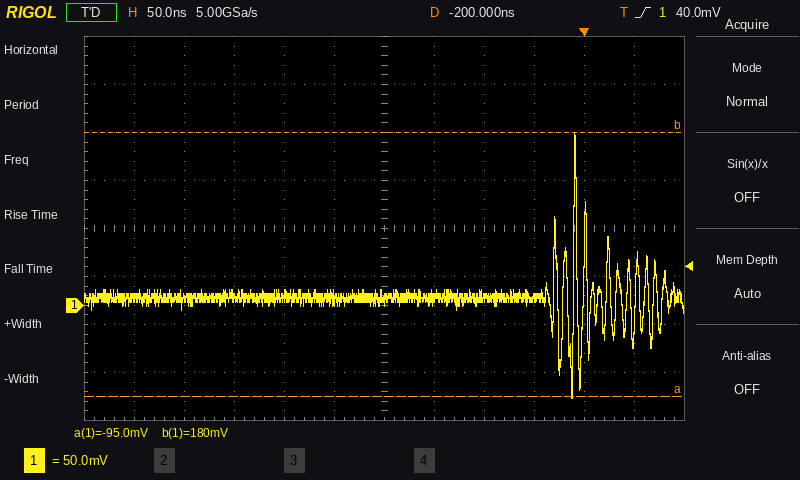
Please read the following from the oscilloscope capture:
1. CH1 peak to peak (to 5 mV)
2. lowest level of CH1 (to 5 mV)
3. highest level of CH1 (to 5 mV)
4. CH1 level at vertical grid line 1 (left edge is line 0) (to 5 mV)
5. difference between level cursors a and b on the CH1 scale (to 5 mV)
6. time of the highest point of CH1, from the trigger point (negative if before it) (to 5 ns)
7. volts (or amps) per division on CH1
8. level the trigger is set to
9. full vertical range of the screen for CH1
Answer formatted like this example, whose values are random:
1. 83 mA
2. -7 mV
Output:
1. 275 mV
2. -95 mV
3. 180 mV
4. 10 mV
5. 275 mV
6. -10 ns
7. 50 mV
8. 40.0 mV
9. 400 mV
